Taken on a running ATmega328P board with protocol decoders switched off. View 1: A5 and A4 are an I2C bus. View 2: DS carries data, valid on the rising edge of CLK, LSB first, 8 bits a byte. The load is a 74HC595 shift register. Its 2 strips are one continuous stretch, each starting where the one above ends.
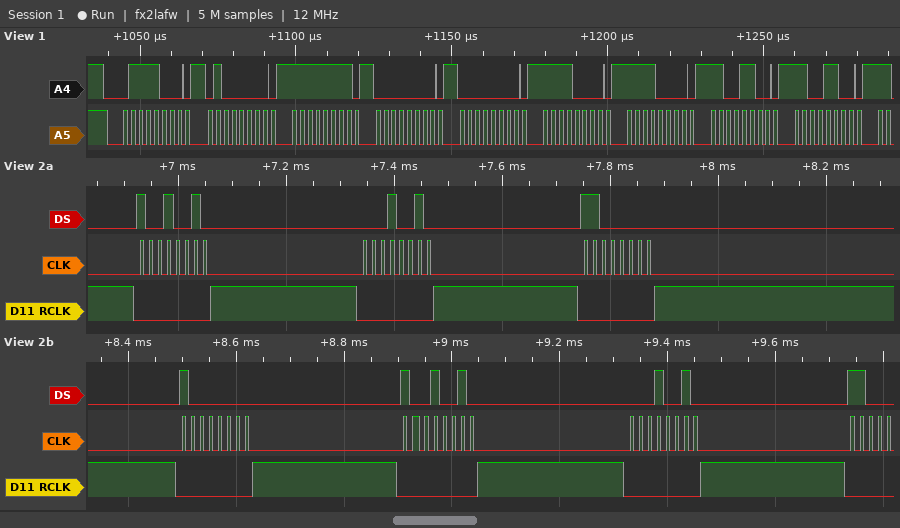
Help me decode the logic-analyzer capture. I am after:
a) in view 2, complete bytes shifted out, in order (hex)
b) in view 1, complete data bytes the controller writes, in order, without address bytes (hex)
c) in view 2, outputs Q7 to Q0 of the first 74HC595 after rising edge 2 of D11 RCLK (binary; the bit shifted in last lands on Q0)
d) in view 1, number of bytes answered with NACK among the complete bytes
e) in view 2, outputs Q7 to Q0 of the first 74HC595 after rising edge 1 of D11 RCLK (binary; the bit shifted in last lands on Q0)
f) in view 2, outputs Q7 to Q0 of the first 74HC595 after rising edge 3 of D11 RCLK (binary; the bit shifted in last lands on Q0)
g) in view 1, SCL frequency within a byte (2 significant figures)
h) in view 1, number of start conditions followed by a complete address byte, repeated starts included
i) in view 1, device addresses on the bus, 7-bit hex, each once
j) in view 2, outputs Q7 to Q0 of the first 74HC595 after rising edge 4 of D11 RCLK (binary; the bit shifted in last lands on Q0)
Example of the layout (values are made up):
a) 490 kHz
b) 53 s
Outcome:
a) 0x49 0x48 0x03 0x01 0x49 0x48
b) 40 FF 00 00 F0 F0 CC CC
c) 00010010
d) 0
e) 10010010
f) 11000000
g) 400 kHz
h) 1
i) 0x3C
j) 10000000
